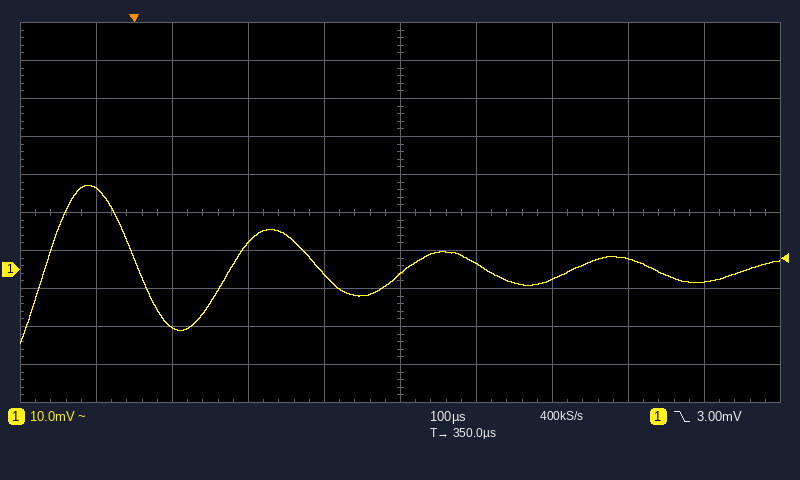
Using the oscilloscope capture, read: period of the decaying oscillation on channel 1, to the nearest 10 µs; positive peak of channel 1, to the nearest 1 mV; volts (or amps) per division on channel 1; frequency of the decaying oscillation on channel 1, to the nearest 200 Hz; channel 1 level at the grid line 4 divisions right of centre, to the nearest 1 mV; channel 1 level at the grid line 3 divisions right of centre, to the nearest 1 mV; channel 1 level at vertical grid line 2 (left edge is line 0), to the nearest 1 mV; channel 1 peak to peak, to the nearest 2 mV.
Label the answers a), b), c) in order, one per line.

a) 230 µs
b) 22 mV
c) 10 mV
d) 4.4 kHz
e) -3 mV
f) 3 mV
g) -15 mV
h) 42 mV
